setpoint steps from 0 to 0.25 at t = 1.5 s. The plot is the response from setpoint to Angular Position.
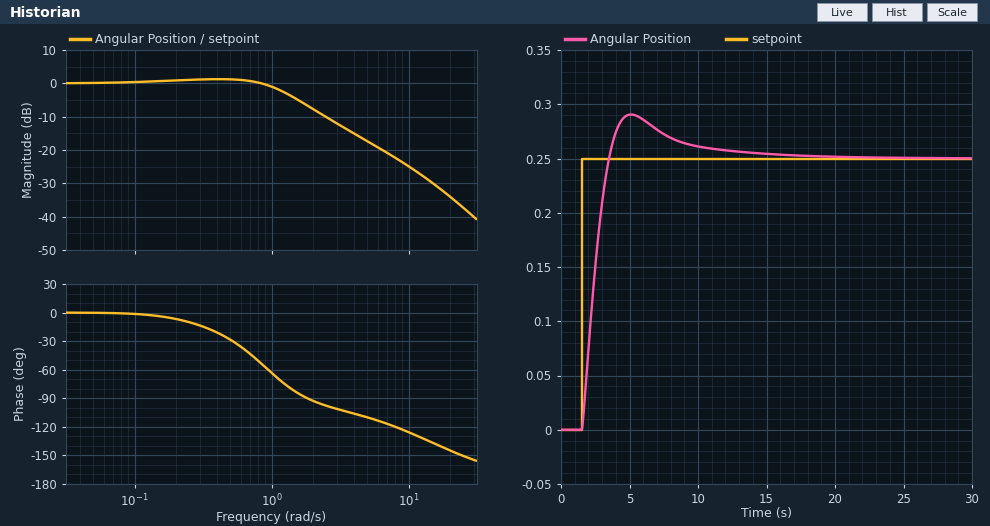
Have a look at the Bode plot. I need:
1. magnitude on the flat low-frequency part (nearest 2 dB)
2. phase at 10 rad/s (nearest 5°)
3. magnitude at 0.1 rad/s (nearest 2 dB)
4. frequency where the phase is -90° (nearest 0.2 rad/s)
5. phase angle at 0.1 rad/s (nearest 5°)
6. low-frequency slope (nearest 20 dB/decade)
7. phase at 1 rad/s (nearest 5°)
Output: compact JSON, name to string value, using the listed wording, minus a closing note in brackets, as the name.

{"magnitude on the flat low-frequency part": "0 dB", "phase at 10 rad/s": "-125°", "magnitude at 0.1 rad/s": "0 dB", "frequency where the phase is -90°": "1.8 rad/s", "phase angle at 0.1 rad/s": "0°", "low-frequency slope": "0 dB/decade", "phase at 1 rad/s": "-65°"}
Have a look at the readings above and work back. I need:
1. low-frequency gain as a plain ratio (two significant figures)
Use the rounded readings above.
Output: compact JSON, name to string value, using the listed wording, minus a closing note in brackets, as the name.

{"low-frequency gain as a plain ratio": "1.0"}
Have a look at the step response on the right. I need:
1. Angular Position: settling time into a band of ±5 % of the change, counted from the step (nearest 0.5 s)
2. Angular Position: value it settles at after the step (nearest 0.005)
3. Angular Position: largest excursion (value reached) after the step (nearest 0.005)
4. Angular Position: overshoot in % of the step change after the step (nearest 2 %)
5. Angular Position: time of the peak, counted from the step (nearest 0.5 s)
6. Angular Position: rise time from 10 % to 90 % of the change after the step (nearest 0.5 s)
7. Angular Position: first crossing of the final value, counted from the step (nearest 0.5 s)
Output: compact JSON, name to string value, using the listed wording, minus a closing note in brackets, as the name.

{"Angular Position: settling time into a band of ±5 % of the change, counted from the step": "8.0 s", "Angular Position: value it settles at after the step": "0.250", "Angular Position: largest excursion (value reached) after the step": "0.290", "Angular Position: overshoot in % of the step change after the step": "16 %", "Angular Position: time of the peak, counted from the step": "3.5 s", "Angular Position: rise time from 10 % to 90 % of the change after the step": "1.5 s", "Angular Position: first crossing of the final value, counted from the step": "2.0 s"}
